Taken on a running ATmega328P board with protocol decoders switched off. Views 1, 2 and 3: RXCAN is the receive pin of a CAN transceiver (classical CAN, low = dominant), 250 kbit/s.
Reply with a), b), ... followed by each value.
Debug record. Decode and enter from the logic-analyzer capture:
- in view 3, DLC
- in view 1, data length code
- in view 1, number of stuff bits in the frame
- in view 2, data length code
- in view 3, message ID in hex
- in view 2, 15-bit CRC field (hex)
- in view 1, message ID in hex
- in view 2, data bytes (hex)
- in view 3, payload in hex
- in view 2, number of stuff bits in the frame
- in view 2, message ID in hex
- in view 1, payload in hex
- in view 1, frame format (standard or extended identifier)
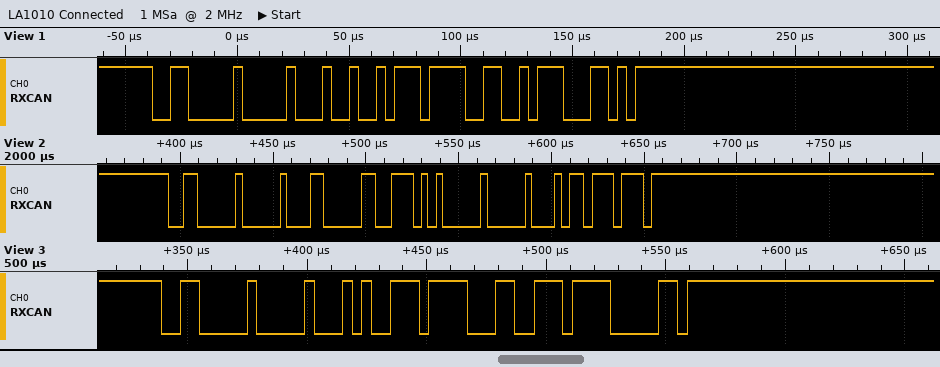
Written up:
a) 2
b) 2
c) 2
d) 3
e) 0x300
f) 0x05BB
g) 0x300
h) 04 EA 00
i) 9D E3
j) 5
k) 0x300
l) 4B BC
m) standard
